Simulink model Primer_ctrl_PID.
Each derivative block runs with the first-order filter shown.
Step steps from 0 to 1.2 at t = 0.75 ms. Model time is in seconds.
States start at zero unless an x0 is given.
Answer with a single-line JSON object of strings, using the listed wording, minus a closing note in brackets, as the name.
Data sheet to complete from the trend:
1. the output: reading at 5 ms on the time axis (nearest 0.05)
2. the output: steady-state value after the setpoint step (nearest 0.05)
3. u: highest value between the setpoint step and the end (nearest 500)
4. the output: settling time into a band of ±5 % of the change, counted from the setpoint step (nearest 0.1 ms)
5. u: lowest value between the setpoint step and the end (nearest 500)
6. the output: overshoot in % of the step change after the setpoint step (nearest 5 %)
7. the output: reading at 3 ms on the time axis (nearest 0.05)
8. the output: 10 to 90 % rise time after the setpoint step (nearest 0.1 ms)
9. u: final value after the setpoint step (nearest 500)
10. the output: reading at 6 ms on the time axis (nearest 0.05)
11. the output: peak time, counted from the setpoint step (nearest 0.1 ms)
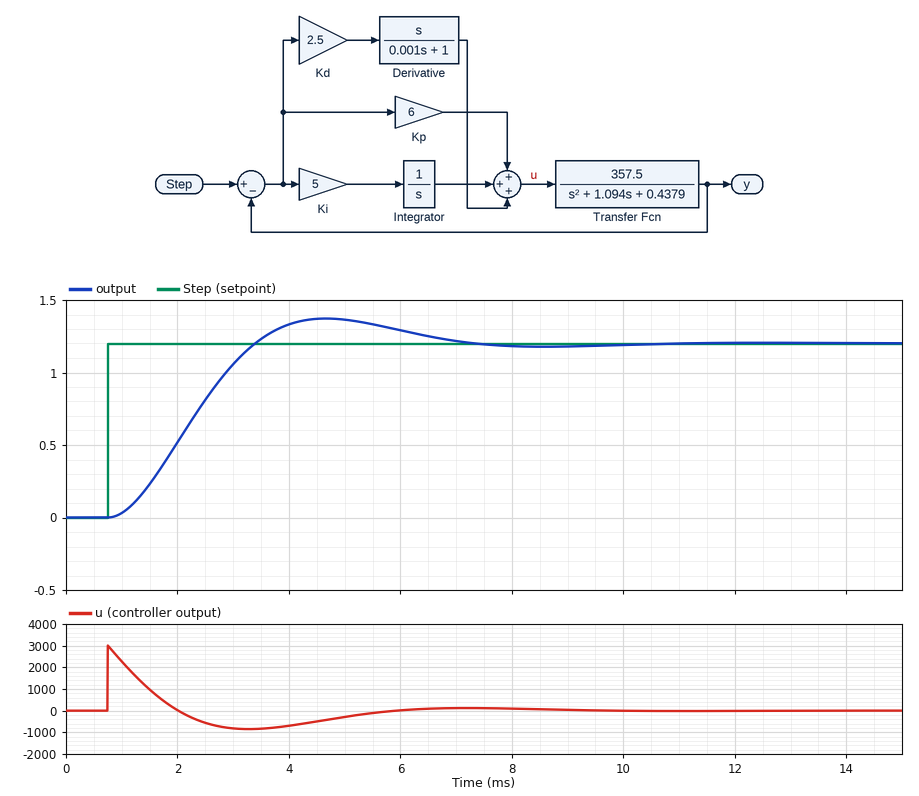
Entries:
{"the output: reading at 5 ms on the time axis": "1.35", "the output: steady-state value after the setpoint step": "1.20", "u: highest value between the setpoint step and the end": "3000", "the output: settling time into a band of ±5 % of the change, counted from the setpoint step": "5.6 ms", "u: lowest value between the setpoint step and the end": "-1000", "the output: overshoot in % of the step change after the setpoint step": "15 %", "the output: reading at 3 ms on the time axis": "1.05", "the output: 10 to 90 % rise time after the setpoint step": "1.8 ms", "u: final value after the setpoint step": "0", "the output: reading at 6 ms on the time axis": "1.30", "the output: peak time, counted from the setpoint step": "3.9 ms"}
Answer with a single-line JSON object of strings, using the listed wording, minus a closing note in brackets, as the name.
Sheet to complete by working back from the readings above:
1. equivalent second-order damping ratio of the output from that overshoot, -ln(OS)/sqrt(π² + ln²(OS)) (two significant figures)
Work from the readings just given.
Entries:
{"equivalent second-order damping ratio of the output from that overshoot, -ln(OS)/sqrt(π² + ln²(OS))": "0.52"}
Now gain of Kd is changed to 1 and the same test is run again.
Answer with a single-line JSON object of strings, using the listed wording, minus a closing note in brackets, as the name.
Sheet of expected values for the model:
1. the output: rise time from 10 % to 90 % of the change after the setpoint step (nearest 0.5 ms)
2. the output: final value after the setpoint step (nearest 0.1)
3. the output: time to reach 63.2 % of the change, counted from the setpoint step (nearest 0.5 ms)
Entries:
{"the output: rise time from 10 % to 90 % of the change after the setpoint step": "4.5 ms", "the output: final value after the setpoint step": "1.2", "the output: time to reach 63.2 % of the change, counted from the setpoint step": "3.0 ms"}
